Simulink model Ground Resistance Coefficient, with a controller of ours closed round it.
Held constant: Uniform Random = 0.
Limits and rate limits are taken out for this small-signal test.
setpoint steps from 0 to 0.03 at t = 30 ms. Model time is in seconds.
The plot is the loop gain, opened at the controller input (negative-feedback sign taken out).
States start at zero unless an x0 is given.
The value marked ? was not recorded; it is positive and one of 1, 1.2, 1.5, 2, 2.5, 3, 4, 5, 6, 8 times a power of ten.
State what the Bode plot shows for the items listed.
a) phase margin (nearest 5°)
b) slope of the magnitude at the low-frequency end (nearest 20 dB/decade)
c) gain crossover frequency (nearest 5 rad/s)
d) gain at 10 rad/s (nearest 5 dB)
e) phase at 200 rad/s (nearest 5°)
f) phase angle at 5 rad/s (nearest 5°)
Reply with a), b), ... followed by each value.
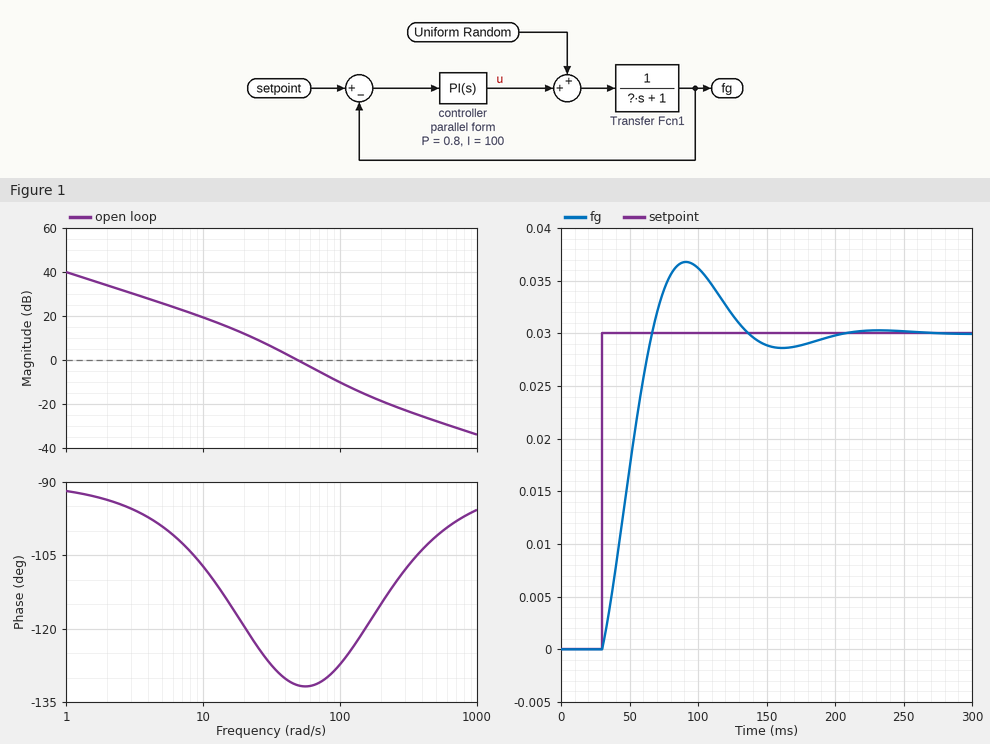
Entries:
a) 50°
b) -20 dB/decade
c) 50 rad/s
d) 20 dB
e) -115°
f) -100°
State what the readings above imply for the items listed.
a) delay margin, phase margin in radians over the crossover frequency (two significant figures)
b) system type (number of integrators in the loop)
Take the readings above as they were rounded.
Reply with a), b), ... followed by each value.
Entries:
a) 0.017 s
b) 1
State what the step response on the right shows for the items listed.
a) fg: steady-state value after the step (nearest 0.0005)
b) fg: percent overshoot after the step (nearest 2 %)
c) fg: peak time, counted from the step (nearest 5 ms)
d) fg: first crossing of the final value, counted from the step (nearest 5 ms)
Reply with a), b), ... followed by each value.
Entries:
a) 0.0300
b) 22 %
c) 60 ms
d) 35 ms
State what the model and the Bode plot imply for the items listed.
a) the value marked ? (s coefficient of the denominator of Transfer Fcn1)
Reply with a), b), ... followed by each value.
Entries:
a) 0.04
